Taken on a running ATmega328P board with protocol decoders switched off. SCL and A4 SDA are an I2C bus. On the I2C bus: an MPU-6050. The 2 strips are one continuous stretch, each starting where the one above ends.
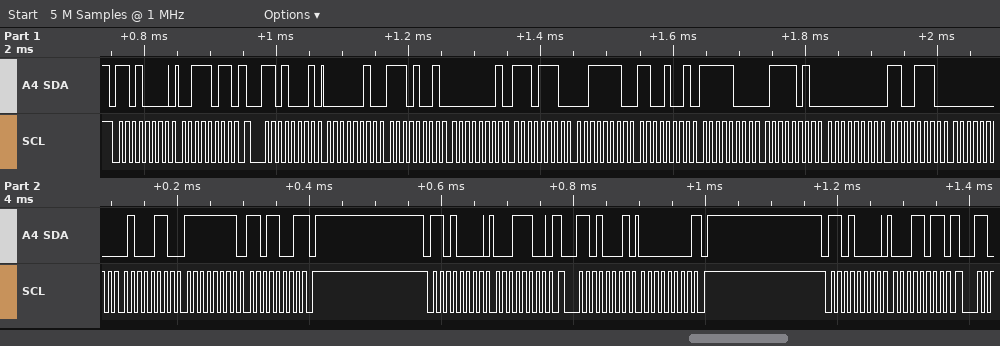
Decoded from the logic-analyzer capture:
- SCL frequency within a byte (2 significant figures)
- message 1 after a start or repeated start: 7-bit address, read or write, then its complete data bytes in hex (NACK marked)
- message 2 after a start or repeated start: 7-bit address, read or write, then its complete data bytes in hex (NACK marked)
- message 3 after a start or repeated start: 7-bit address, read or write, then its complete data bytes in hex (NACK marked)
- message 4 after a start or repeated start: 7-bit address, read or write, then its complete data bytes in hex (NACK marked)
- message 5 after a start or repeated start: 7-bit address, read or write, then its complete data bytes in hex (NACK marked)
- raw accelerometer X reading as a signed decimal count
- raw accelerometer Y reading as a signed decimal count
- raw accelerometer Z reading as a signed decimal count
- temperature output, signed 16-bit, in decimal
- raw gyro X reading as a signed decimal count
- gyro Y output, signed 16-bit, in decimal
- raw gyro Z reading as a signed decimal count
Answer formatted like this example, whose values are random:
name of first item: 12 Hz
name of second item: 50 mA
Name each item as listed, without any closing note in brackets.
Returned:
SCL frequency within a byte: 100 kHz
message 1 after a start or repeated start: 7-bit address, read or write, then its complete data bytes in hex: 0x68 write: 3B
message 2 after a start or repeated start: 7-bit address, read or write, then its complete data bytes in hex: 0x68 read: 02 E9 01 EE 3E C9 F8 7A 00 CE 00 46 FF D9 NACK
message 3 after a start or repeated start: 7-bit address, read or write, then its complete data bytes in hex: 0x68 write: 1C
message 4 after a start or repeated start: 7-bit address, read or write, then its complete data bytes in hex: 0x68 read: 00 NACK
message 5 after a start or repeated start: 7-bit address, read or write, then its complete data bytes in hex: 0x68 write: 1B
raw accelerometer X reading as a signed decimal count: 745
raw accelerometer Y reading as a signed decimal count: 494
raw accelerometer Z reading as a signed decimal count: 16073
temperature output, signed 16-bit, in decimal: -1926
raw gyro X reading as a signed decimal count: 206
gyro Y output, signed 16-bit, in decimal: 70
raw gyro Z reading as a signed decimal count: -39
